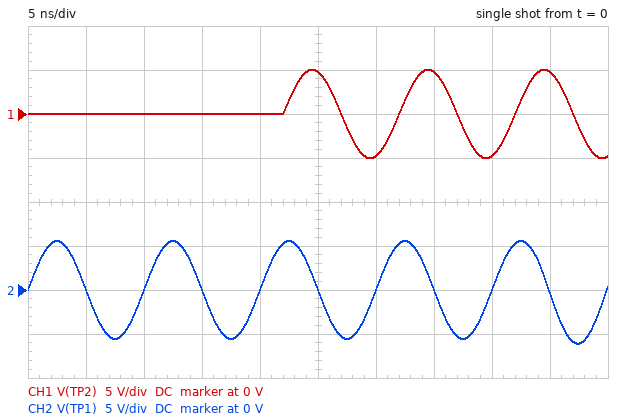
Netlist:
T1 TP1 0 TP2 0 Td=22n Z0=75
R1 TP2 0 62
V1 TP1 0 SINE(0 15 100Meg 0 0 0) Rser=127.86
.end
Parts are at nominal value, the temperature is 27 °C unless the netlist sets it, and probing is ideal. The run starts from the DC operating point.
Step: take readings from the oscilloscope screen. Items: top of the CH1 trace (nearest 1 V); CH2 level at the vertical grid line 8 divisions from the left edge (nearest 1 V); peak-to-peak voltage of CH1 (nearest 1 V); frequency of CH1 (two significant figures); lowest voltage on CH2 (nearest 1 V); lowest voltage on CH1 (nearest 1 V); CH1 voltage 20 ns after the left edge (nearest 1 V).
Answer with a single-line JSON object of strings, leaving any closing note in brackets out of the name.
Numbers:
{"top of the CH1 trace": "5 V", "CH2 level at the vertical grid line 8 divisions from the left edge": "0 V", "peak-to-peak voltage of CH1": "10 V", "frequency of CH1": "100 MHz", "lowest voltage on CH2": "-6 V", "lowest voltage on CH1": "-5 V", "CH1 voltage 20 ns after the left edge": "0 V"}
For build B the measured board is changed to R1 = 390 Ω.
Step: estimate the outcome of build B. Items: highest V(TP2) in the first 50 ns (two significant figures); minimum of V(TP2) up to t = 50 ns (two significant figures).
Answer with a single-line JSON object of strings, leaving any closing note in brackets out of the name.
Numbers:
{"highest V(TP2) in the first 50 ns": "9.3 V", "minimum of V(TP2) up to t = 50 ns": "-9.3 V"}
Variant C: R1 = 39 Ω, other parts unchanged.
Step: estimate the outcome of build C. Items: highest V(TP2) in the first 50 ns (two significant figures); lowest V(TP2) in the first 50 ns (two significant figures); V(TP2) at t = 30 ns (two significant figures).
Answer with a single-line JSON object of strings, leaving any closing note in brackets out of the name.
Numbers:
{"highest V(TP2) in the first 50 ns": "3.8 V", "lowest V(TP2) in the first 50 ns": "-3.8 V", "V(TP2) at t = 30 ns": "-3.6 V"}
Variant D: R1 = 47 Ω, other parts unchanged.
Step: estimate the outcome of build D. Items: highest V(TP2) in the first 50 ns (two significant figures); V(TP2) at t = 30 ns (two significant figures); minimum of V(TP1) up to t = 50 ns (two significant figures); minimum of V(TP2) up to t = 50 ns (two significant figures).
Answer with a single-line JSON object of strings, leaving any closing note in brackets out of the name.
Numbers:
{"highest V(TP2) in the first 50 ns": "4.3 V", "V(TP2) at t = 30 ns": "-4.1 V", "minimum of V(TP1) up to t = 50 ns": "-6.9 V", "minimum of V(TP2) up to t = 50 ns": "-4.3 V"}
